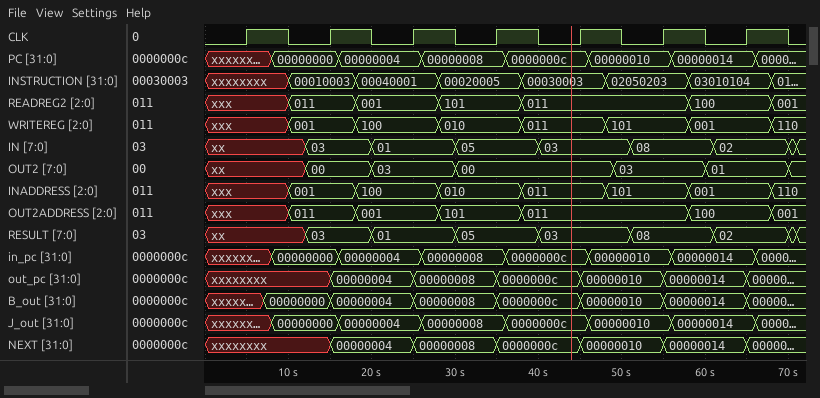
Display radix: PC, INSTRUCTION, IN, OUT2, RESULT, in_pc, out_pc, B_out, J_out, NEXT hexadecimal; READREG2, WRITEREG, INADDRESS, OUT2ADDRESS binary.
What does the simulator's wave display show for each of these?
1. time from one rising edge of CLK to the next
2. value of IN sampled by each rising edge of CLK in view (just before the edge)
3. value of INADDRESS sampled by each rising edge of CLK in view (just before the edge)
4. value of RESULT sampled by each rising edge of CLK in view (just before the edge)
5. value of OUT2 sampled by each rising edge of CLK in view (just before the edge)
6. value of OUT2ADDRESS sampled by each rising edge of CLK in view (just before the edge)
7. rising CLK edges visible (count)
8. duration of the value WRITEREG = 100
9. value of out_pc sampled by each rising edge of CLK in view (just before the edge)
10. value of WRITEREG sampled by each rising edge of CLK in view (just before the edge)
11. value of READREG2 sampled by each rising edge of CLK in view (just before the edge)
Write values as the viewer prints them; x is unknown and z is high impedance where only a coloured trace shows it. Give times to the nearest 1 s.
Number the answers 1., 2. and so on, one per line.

1. 10 s
2. xx, 03, 01, 05, 03, 08, 02
3. xxx, 001, 100, 010, 011, 101, 001
4. xx, 03, 01, 05, 03, 08, 02
5. xx, 00, 03, 00, 00, 03, 01
6. xxx, 011, 001, 101, 011, 011, 100
7. 7
8. 10 s
9. xxxxxxxx, xxxxxxxx, 00000004, 00000008, 0000000c, 00000010, 00000014
10. xxx, 001, 100, 010, 011, 101, 001
11. xxx, 011, 001, 101, 011, 011, 100
